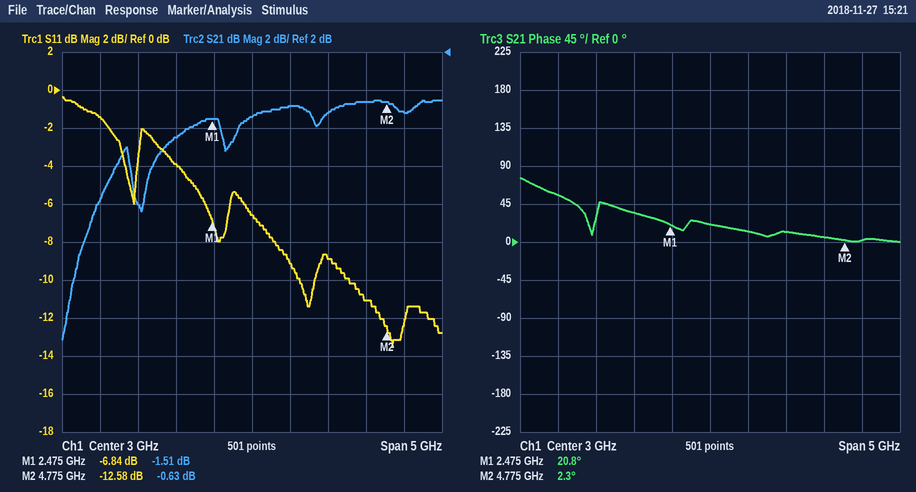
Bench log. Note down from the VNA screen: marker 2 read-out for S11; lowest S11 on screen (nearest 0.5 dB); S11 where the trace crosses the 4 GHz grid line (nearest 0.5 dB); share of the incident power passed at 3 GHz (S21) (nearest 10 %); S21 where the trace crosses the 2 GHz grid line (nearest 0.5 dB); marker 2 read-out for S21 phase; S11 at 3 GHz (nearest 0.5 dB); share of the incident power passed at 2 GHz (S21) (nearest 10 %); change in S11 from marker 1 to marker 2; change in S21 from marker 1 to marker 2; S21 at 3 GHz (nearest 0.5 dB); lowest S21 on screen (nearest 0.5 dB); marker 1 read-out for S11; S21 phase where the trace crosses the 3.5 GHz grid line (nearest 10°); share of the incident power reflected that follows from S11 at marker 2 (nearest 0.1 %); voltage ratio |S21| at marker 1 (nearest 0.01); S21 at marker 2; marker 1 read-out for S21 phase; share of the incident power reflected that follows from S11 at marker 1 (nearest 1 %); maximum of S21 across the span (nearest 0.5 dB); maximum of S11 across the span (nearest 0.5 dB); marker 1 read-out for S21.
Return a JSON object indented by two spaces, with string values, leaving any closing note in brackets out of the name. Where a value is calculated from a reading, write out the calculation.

{
  "marker 2 read-out for S11": "-12.58 dB",
  "lowest S11 on screen": "-13.5 dB",
  "S11 where the trace crosses the 4 GHz grid line": "-9.0 dB",
  "share of the incident power passed at 3 GHz (S21)": "10^(-1.5/10) ≈ 70.8 %, so 70 % to the nearest 10 %",
  "S21 where the trace crosses the 2 GHz grid line": "-2.5 dB",
  "marker 2 read-out for S21 phase": "2.3°",
  "S11 at 3 GHz": "-6.5 dB",
  "share of the incident power passed at 2 GHz (S21)": "10^(-2.5/10) ≈ 56.2 %, so 60 % to the nearest 10 %",
  "change in S11 from marker 1 to marker 2": "-12.58 − (-6.84) = -5.74 dB",
  "change in S21 from marker 1 to marker 2": "-0.63 − (-1.51) = 0.88 dB",
  "S21 at 3 GHz": "-1.5 dB",
  "lowest S21 on screen": "-13.0 dB",
  "marker 1 read-out for S11": "-6.84 dB",
  "S21 phase where the trace crosses the 3.5 GHz grid line": "10°",
  "share of the incident power reflected that follows from S11 at marker 2": "10^(-12.58/10) ≈ 5.5 %",
  "voltage ratio |S21| at marker 1": "10^(-1.51/20) ≈ 0.84",
  "S21 at marker 2": "-0.63 dB",
  "marker 1 read-out for S21 phase": "20.8°",
  "share of the incident power reflected that follows from S11 at marker 1": "10^(-6.84/10) ≈ 21 %",
  "maximum of S21 across the span": "-0.5 dB",
  "maximum of S11 across the span": "-0.5 dB",
  "marker 1 read-out for S21": "-1.51 dB"
}
